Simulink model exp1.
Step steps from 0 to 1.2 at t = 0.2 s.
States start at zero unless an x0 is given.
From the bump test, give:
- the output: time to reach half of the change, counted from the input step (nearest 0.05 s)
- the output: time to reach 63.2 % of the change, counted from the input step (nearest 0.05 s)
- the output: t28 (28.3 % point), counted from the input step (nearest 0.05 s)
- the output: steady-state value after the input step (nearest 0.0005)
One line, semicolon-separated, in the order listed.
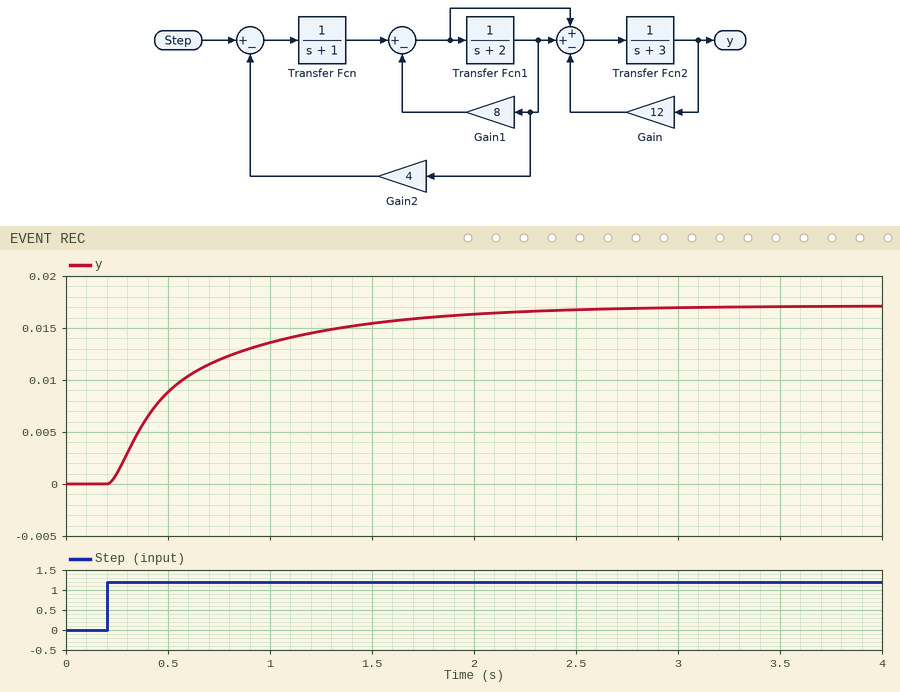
0.30 s; 0.45 s; 0.15 s; 0.0170
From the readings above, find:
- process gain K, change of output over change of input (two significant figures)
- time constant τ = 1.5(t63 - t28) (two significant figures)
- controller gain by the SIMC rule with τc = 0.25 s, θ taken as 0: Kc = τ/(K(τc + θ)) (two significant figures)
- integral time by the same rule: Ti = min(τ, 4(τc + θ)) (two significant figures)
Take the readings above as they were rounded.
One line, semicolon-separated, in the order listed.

0.014; 0.45 s; 130; 0.45 s
